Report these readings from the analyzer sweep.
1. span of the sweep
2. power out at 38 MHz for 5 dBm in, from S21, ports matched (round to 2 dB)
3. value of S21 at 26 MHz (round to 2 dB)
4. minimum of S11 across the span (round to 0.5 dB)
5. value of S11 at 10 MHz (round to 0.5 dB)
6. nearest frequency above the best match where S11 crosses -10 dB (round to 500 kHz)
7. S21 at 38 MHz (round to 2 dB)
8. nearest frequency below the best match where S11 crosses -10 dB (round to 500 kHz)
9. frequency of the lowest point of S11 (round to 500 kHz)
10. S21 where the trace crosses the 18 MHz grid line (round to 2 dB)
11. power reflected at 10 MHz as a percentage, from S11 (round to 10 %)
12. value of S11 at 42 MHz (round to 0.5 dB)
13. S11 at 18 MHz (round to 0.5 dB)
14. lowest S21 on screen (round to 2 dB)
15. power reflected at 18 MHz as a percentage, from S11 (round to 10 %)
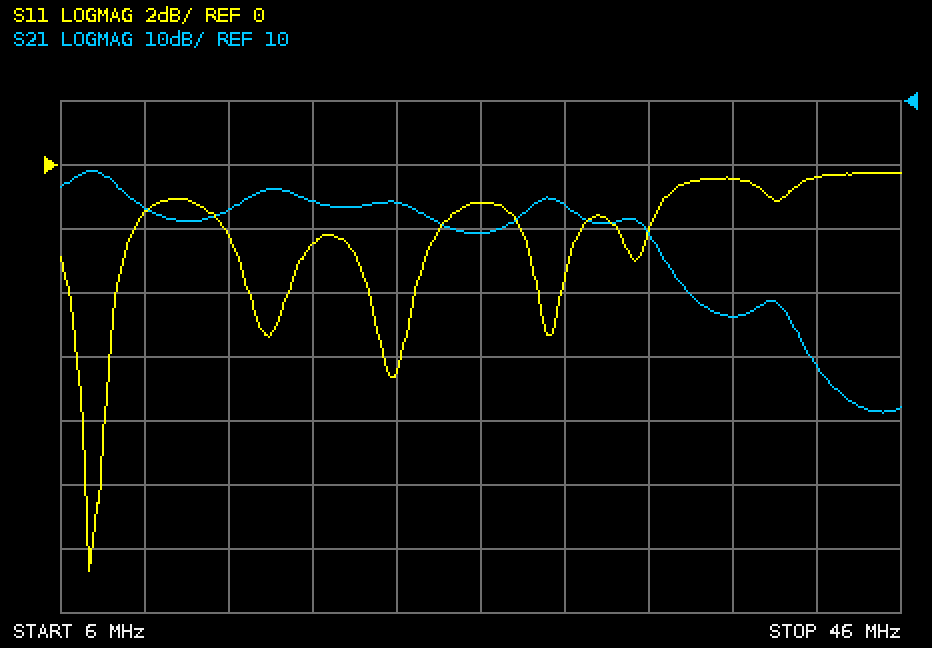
40 MHz
-18 dBm
-10 dB
-12.5 dB
-1.5 dB
8.0 MHz
-24 dB
7.0 MHz
7.5 MHz
-6 dB
70 %
-0.5 dB
-2.5 dB
-38 dB
60 %
